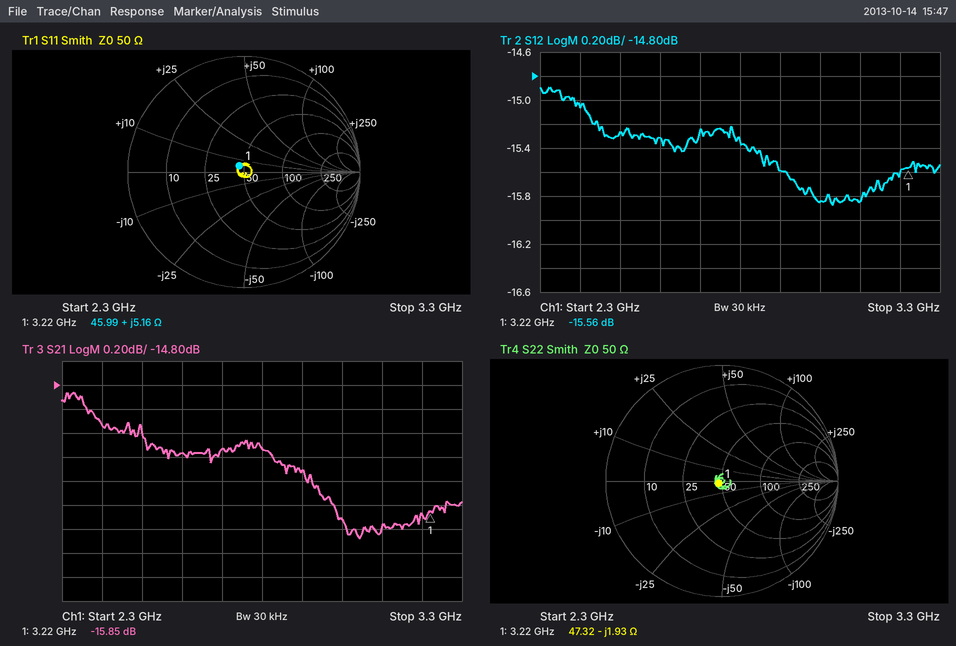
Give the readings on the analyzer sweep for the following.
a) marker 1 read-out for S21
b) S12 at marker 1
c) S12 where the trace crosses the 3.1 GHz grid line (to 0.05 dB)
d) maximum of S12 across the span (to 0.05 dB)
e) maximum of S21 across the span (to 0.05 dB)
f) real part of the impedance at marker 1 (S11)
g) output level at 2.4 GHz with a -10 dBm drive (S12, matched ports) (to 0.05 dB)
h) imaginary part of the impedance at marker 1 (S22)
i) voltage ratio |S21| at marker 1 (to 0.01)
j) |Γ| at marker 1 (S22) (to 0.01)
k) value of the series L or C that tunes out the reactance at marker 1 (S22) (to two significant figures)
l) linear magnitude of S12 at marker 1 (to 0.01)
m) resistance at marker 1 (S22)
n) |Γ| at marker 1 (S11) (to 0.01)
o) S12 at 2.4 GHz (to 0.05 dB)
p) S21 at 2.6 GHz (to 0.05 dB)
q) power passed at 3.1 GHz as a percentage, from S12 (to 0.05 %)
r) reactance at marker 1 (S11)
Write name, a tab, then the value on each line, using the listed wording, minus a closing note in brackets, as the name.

marker 1 read-out for S21	-15.85 dB
S12 at marker 1	-15.56 dB
S12 where the trace crosses the 3.1 GHz grid line	-15.85 dB
maximum of S12 across the span	-14.90 dB
maximum of S21 across the span	-14.85 dB
real part of the impedance at marker 1	45.99 Ω
output level at 2.4 GHz with a -10 dBm drive (S12, matched ports)	-25.05 dBm
imaginary part of the impedance at marker 1	-1.93 Ω
voltage ratio |S21| at marker 1	0.16
|Γ| at marker 1 (S22)	0.03
value of the series L or C that tunes out the reactance at marker 1 (S22)	95 pH
linear magnitude of S12 at marker 1	0.17
resistance at marker 1	47.32 Ω
|Γ| at marker 1 (S11)	0.07
S12 at 2.4 GHz	-15.05 dB
S21 at 2.6 GHz	-15.35 dB
power passed at 3.1 GHz as a percentage, from S12	2.60 %
reactance at marker 1	+5.16 Ω
